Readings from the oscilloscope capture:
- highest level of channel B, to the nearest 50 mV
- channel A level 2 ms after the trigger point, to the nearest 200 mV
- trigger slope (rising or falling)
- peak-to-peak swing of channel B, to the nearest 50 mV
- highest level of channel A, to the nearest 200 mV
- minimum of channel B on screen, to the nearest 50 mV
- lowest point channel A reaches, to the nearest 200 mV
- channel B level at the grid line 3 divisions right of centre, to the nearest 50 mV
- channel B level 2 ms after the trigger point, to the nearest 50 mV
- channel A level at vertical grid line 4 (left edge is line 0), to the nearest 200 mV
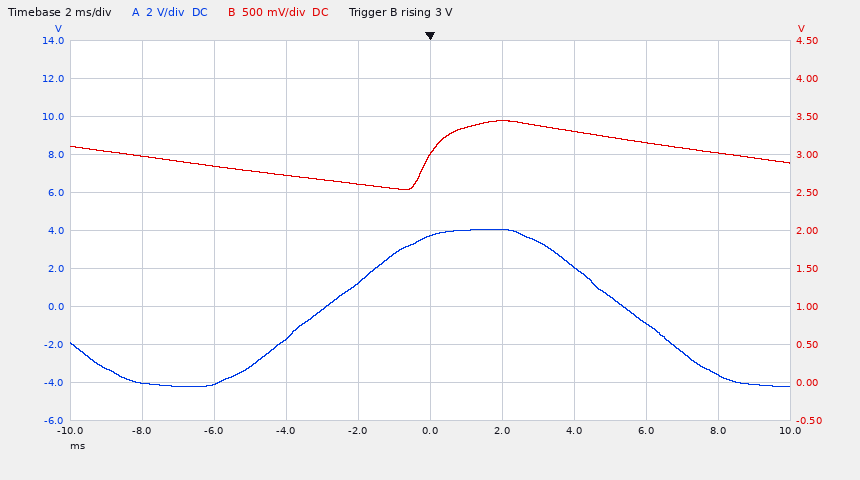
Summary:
3.45 V
4.0 V
rising
900 mV
4.0 V
2.55 V
-4.2 V
3.15 V
3.45 V
1.2 V
